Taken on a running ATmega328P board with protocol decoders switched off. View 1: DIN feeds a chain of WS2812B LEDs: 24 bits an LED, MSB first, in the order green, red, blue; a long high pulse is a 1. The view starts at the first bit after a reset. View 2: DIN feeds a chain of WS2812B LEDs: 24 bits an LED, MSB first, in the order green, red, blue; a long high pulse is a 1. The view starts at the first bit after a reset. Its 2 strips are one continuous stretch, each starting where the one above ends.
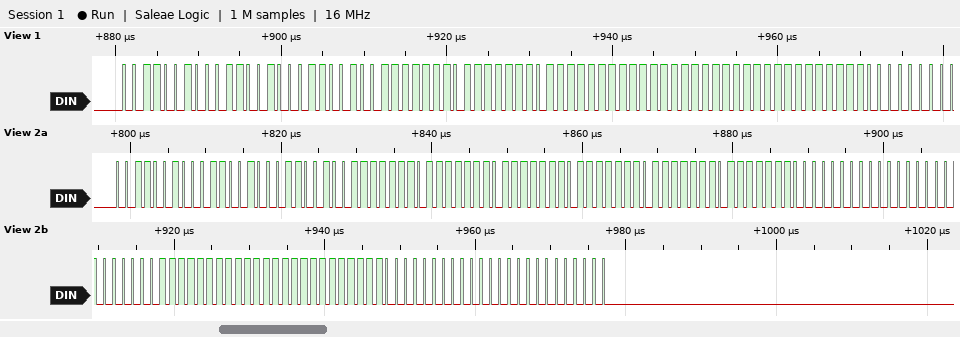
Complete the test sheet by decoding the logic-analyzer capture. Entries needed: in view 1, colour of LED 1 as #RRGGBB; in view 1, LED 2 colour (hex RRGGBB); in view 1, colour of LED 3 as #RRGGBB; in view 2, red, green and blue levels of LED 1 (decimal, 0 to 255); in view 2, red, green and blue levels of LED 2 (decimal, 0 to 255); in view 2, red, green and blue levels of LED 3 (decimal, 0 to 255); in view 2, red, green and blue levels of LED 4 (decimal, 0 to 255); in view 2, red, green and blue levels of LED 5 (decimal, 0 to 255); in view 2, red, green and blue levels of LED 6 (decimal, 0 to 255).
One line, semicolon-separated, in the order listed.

#323232; #7F7F7F; #FFFFFF; 50, 50, 50; 127, 127, 127; 127, 127, 127; 0, 0, 0; 255, 255, 255; 0, 0, 0
